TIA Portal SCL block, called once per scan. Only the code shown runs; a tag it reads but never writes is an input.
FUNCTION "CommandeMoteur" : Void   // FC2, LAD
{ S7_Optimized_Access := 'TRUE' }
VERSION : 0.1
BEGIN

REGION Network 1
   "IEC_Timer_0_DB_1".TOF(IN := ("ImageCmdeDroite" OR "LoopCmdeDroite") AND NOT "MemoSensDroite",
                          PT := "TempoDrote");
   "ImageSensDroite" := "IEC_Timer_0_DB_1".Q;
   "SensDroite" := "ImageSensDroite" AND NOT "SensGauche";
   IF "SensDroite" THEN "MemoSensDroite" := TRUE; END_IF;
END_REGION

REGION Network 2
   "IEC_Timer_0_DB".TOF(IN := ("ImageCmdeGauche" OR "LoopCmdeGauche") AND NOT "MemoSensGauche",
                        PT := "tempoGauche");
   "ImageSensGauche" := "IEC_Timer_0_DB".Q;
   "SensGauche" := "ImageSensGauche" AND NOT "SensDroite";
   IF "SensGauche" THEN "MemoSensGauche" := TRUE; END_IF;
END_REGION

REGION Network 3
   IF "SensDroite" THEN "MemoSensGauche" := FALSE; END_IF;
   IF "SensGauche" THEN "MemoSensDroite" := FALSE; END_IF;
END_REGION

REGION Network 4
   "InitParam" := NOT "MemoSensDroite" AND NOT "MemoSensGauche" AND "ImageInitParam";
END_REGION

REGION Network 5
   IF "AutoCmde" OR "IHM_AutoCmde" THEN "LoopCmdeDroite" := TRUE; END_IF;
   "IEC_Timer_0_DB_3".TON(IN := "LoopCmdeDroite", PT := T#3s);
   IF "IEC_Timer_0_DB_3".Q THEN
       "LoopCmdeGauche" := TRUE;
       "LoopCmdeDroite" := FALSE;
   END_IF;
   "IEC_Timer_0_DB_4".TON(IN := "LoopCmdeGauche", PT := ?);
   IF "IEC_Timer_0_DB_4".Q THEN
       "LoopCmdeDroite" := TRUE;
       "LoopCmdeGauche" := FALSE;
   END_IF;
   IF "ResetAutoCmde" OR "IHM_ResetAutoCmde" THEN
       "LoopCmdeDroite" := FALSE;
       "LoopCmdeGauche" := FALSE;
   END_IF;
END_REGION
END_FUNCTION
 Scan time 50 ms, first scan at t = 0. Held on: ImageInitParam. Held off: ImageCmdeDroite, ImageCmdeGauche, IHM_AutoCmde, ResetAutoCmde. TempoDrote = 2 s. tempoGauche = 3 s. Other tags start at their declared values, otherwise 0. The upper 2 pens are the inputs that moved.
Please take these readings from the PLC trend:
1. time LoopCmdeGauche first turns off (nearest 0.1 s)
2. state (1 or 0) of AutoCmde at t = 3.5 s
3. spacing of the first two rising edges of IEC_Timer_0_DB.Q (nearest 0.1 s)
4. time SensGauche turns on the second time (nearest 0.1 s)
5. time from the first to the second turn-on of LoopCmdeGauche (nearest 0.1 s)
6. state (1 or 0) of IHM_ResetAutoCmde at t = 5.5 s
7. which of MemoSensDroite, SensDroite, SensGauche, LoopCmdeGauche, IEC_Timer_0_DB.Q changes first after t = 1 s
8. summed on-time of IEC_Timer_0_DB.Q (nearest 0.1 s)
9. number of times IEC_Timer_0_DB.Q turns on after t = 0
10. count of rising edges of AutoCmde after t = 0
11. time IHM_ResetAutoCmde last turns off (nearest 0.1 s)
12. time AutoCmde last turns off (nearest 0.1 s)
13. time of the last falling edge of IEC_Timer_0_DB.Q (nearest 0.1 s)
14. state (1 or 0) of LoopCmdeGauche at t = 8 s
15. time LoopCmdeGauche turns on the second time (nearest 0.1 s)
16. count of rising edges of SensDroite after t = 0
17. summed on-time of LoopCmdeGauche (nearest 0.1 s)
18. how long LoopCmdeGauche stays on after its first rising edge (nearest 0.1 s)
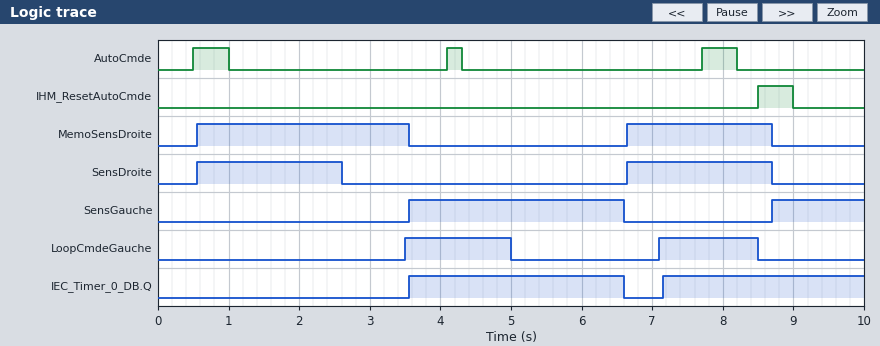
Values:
5.0 s
0
3.6 s
8.7 s
3.6 s
0
SensDroite
5.9 s
2
3
9.0 s
8.2 s
6.6 s
1
7.1 s
2
2.9 s
1.5 s
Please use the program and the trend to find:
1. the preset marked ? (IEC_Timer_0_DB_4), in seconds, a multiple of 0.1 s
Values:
1.5 s
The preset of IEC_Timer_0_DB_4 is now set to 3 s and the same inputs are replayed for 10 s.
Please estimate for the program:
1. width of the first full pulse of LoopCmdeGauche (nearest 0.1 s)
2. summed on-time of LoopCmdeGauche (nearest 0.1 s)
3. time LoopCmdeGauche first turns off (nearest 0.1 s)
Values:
3.0 s
4.4 s
6.5 s
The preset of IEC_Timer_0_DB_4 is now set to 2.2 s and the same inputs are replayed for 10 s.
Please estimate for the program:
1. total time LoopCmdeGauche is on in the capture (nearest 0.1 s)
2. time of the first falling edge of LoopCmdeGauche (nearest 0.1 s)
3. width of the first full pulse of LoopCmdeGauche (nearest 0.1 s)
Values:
3.6 s
5.7 s
2.2 s
